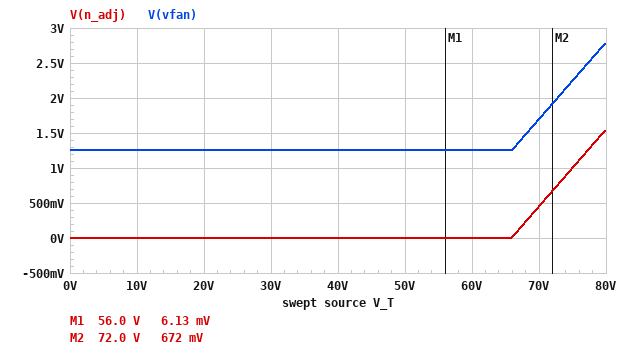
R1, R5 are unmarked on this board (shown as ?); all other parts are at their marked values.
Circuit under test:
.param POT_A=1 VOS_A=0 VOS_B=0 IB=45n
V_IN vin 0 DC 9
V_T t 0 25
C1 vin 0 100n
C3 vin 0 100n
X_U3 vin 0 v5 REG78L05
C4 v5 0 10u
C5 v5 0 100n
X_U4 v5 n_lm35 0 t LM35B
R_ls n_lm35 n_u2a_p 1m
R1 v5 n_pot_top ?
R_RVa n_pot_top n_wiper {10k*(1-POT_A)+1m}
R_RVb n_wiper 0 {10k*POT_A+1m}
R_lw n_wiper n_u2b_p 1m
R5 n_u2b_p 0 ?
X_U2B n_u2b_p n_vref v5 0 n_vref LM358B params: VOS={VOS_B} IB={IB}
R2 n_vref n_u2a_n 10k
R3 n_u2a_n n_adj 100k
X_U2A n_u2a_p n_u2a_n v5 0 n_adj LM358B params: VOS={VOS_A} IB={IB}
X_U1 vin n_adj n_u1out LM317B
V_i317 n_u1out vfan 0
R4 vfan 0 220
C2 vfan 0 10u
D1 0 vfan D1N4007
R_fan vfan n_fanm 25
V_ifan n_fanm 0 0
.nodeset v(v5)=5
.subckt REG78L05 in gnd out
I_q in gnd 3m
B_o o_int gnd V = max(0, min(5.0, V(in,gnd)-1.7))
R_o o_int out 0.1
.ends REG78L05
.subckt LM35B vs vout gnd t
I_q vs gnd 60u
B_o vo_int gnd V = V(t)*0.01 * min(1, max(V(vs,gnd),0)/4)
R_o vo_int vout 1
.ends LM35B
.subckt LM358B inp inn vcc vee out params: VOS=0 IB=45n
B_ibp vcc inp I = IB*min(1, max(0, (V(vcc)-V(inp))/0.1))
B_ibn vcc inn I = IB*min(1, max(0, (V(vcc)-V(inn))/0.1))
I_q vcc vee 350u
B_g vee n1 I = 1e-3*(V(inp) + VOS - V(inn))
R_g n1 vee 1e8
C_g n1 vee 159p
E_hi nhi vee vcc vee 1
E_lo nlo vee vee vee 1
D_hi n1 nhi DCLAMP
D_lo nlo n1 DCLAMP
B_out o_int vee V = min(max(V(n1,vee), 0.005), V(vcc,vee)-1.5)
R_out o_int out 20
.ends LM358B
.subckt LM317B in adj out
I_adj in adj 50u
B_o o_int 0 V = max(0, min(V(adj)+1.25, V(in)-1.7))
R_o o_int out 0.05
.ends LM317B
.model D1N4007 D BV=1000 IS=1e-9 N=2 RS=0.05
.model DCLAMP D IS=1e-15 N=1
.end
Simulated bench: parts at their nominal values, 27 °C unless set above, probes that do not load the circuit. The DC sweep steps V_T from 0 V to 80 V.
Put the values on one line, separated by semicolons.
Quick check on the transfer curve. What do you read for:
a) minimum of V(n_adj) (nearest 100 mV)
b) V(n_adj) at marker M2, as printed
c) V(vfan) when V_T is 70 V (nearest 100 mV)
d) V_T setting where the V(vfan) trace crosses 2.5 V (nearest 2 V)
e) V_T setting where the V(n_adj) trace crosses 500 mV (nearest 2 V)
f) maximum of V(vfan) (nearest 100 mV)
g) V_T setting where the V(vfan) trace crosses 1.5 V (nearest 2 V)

0 V; 672 mV; 1.7 V; 78 V; 70 V; 2.8 V; 68 V
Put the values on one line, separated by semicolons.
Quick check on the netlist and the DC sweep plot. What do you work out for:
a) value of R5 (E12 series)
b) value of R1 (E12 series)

39 kΩ; 47 kΩ
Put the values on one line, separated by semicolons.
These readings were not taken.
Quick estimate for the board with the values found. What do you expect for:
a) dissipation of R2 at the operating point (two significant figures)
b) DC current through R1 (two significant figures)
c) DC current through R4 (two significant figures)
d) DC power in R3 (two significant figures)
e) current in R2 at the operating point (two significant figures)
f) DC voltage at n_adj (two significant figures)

420 nW; 91 µA; 5.7 mA; 4.3 µW; 6.5 µA; 6.1 mV
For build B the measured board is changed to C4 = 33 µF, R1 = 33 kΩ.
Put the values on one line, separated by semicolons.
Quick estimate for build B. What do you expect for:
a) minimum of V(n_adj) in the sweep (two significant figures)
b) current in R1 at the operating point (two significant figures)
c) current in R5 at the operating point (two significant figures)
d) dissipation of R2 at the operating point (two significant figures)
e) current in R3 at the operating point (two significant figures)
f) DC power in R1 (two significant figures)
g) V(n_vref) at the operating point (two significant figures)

6.2 mV; 120 µA; 25 µA; 760 nW; 8.8 µA; 490 µW; 970 mV
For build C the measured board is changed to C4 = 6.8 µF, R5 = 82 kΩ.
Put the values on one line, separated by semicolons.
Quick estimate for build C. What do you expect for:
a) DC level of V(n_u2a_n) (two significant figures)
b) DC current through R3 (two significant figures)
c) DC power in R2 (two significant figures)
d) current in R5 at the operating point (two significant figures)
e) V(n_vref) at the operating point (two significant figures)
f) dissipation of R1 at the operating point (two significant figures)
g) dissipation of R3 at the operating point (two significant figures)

730 mV; 7.2 µA; 510 nW; 9.7 µA; 800 mV; 380 µW; 5.2 µW
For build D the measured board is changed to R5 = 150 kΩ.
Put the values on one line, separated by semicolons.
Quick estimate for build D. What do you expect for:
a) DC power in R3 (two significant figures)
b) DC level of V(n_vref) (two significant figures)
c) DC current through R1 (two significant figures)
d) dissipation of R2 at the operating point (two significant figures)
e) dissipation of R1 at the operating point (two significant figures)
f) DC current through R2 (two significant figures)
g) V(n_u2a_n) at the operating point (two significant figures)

5.6 µW; 830 mV; 89 µA; 560 nW; 370 µW; 7.5 µA; 760 mV
